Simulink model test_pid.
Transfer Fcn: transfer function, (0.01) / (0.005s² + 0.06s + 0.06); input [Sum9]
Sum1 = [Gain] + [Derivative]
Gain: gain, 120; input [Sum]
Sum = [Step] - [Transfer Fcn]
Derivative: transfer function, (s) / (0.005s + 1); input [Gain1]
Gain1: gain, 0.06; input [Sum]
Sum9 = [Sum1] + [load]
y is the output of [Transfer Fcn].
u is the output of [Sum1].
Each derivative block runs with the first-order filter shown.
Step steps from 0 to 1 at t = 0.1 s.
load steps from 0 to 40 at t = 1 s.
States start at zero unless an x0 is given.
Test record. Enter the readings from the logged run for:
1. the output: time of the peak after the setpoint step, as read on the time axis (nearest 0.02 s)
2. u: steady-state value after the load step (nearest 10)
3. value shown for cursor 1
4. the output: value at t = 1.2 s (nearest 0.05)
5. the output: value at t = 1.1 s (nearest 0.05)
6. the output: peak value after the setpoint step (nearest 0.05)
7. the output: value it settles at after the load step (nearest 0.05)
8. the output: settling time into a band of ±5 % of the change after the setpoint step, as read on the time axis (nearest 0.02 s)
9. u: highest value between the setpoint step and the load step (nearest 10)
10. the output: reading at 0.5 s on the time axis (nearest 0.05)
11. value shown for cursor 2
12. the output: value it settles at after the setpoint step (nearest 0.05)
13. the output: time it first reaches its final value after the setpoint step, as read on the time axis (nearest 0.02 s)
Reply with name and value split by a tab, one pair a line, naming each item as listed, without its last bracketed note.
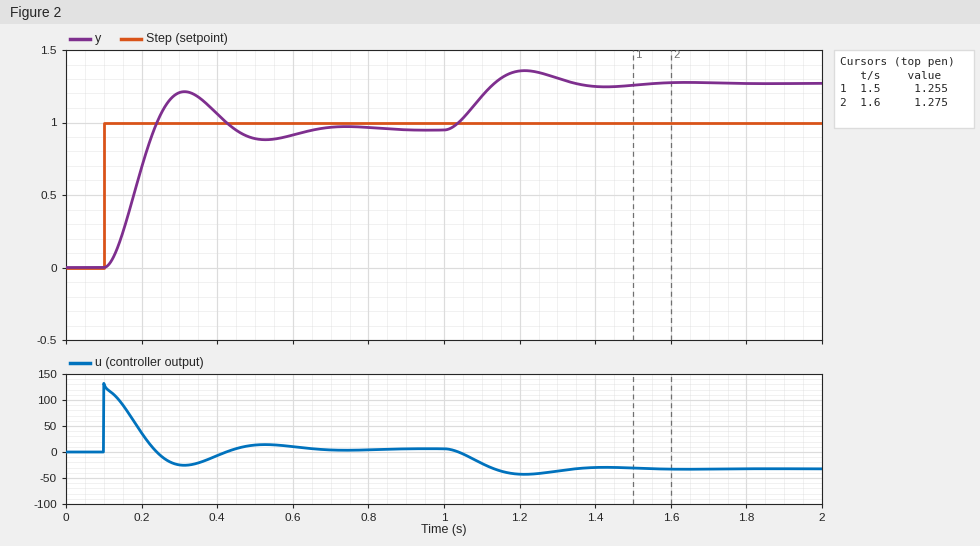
the output: time of the peak after the setpoint step, as read on the time axis	0.32 s
u: steady-state value after the load step	-30
value shown for cursor 1	1.255
the output: value at t = 1.2 s	1.35
the output: value at t = 1.1 s	1.20
the output: peak value after the setpoint step	1.20
the output: value it settles at after the load step	1.25
the output: settling time into a band of ±5 % of the change after the setpoint step, as read on the time axis	0.58 s
u: highest value between the setpoint step and the load step	130
the output: reading at 0.5 s on the time axis	0.90
value shown for cursor 2	1.275
the output: value it settles at after the setpoint step	0.95
the output: time it first reaches its final value after the setpoint step, as read on the time axis	0.24 s
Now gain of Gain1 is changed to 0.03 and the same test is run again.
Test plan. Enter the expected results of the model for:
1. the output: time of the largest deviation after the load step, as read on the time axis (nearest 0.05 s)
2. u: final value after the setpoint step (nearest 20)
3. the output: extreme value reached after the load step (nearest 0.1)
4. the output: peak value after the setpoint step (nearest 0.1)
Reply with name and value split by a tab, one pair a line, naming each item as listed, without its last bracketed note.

the output: time of the largest deviation after the load step, as read on the time axis	1.20 s
u: final value after the setpoint step	0
the output: extreme value reached after the load step	1.4
the output: peak value after the setpoint step	1.2
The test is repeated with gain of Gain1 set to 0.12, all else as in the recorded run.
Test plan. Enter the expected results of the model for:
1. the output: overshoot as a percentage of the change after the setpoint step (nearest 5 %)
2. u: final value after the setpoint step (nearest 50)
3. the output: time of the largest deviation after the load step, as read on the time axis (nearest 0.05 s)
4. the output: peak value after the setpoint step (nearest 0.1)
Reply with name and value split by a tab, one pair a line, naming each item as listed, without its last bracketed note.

the output: overshoot as a percentage of the change after the setpoint step	25 %
u: final value after the setpoint step	0
the output: time of the largest deviation after the load step, as read on the time axis	1.20 s
the output: peak value after the setpoint step	1.2
